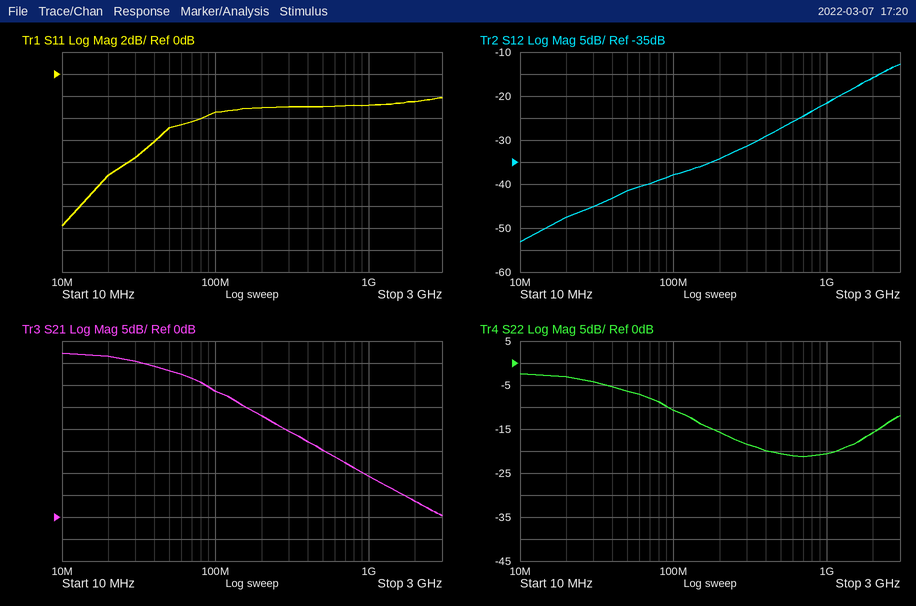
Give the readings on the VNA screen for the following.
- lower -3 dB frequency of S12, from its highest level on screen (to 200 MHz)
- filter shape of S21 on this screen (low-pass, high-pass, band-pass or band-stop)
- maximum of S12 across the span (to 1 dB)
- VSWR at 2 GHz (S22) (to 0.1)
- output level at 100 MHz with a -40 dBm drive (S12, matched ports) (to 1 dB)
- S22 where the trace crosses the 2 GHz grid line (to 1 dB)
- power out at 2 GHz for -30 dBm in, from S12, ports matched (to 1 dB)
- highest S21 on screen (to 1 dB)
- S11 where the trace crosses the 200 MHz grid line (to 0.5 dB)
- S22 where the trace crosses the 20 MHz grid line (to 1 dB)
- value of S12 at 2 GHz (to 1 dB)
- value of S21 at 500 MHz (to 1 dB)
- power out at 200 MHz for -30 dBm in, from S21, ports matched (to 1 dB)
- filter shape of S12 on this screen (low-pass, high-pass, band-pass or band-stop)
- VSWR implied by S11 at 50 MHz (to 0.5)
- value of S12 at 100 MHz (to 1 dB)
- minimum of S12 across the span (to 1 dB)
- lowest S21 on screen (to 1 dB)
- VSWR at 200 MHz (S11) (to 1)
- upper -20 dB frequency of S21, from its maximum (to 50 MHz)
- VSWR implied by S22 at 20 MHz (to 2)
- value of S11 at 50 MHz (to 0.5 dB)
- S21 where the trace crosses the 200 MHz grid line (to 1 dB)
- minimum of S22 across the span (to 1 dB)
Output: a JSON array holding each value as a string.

["2.0 GHz", "low-pass", "-13 dB", "1.4", "-78 dBm", "-16 dB", "-46 dBm", "37 dB", "-3.0 dB", "-3 dB", "-16 dB", "15 dB", "-7 dBm", "high-pass", "3.5", "-38 dB", "-53 dB", "0 dB", "6", "400 MHz", "6", "-5.0 dB", "23 dB", "-21 dB"]
